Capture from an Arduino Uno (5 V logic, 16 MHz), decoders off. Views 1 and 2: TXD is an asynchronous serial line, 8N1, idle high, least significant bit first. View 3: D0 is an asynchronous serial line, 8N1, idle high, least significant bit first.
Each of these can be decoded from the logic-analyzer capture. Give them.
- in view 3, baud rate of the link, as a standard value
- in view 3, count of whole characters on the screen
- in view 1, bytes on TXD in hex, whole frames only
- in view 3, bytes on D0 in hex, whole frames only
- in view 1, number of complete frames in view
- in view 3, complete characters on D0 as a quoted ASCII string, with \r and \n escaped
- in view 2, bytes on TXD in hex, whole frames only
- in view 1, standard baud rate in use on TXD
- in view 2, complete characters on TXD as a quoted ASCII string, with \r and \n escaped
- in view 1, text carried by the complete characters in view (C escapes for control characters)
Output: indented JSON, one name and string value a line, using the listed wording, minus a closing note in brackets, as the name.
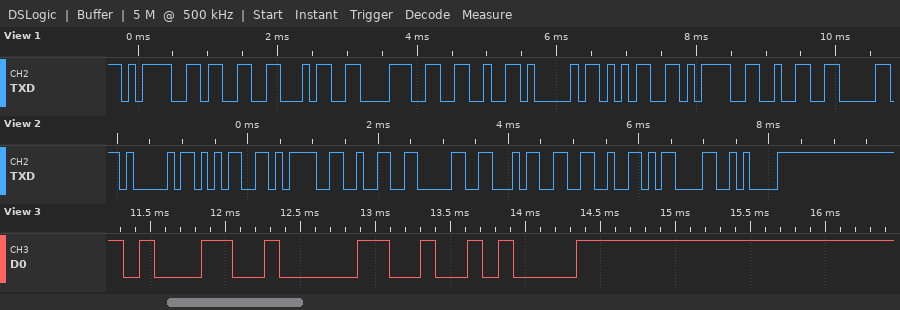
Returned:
{
  "in view 3, baud rate of the link, as a standard value": "9600 baud",
  "in view 3, count of whole characters on the screen": "3",
  "in view 1, bytes on TXD in hex, whole frames only": "3D 33 34 38 26 41 35 3D 32",
  "in view 3, bytes on D0 in hex, whole frames only": "31 30 0A",
  "in view 1, number of complete frames in view": "9",
  "in view 3, complete characters on D0 as a quoted ASCII string, with \\r and \\n escaped": "\"10\\n\"",
  "in view 2, bytes on TXD in hex, whole frames only": "41 35 3D 32 30 34 26 0D 0A",
  "in view 1, standard baud rate in use on TXD": "9600 baud",
  "in view 2, complete characters on TXD as a quoted ASCII string, with \\r and \\n escaped": "\"A5=204&\\r\\n\"",
  "in view 1, text carried by the complete characters in view": "\"=348&A5=2\""
}
